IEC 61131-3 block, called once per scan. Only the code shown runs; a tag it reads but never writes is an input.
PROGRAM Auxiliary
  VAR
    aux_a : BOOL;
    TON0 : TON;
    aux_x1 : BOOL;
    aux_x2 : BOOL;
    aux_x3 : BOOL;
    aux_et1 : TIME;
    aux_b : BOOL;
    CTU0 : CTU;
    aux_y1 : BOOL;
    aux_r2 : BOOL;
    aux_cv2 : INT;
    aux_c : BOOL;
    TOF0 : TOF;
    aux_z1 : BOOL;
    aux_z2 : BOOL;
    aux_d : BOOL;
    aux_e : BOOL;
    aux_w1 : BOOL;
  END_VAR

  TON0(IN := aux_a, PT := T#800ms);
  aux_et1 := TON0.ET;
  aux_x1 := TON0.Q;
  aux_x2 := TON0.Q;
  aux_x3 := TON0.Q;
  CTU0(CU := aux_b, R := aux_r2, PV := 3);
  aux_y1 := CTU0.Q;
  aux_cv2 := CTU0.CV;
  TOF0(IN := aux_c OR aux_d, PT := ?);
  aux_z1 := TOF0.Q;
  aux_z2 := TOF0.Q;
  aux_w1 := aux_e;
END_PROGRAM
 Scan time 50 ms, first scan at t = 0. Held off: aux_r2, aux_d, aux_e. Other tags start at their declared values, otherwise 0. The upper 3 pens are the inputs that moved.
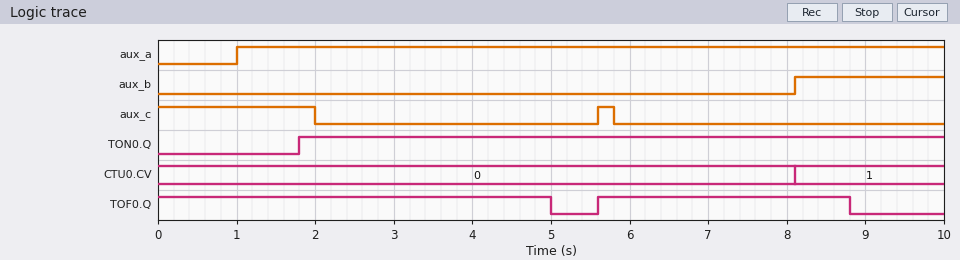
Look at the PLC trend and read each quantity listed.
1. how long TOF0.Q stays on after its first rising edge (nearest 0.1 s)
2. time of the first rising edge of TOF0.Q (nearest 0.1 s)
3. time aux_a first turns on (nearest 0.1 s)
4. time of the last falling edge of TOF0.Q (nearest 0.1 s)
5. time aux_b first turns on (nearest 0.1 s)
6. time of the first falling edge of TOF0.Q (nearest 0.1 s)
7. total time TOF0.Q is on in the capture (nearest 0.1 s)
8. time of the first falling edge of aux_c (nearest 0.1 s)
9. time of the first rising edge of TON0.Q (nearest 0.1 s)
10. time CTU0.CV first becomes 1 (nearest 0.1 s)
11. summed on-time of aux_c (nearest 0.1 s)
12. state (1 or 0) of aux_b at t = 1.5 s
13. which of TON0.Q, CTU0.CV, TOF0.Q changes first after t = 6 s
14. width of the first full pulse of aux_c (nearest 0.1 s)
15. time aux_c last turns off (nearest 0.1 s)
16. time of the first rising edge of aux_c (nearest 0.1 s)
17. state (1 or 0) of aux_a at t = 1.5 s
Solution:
3.2 s
5.6 s
1.0 s
8.8 s
8.1 s
5.0 s
8.2 s
2.0 s
1.8 s
8.1 s
2.2 s
0
CTU0.CV
0.2 s
5.8 s
5.6 s
1
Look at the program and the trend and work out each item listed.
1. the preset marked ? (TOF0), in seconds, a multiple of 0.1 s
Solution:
3.0 s
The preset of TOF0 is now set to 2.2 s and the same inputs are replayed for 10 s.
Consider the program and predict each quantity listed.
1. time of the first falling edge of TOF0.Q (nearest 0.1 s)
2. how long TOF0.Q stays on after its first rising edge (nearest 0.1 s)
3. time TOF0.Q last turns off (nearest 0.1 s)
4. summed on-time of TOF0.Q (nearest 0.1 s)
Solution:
4.2 s
2.4 s
8.0 s
6.6 s
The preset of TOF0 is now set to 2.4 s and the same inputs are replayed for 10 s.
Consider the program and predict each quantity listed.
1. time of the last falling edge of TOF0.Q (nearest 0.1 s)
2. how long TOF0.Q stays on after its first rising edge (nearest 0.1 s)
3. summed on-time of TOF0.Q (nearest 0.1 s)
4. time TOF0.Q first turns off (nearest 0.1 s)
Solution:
8.2 s
2.6 s
7.0 s
4.4 s
